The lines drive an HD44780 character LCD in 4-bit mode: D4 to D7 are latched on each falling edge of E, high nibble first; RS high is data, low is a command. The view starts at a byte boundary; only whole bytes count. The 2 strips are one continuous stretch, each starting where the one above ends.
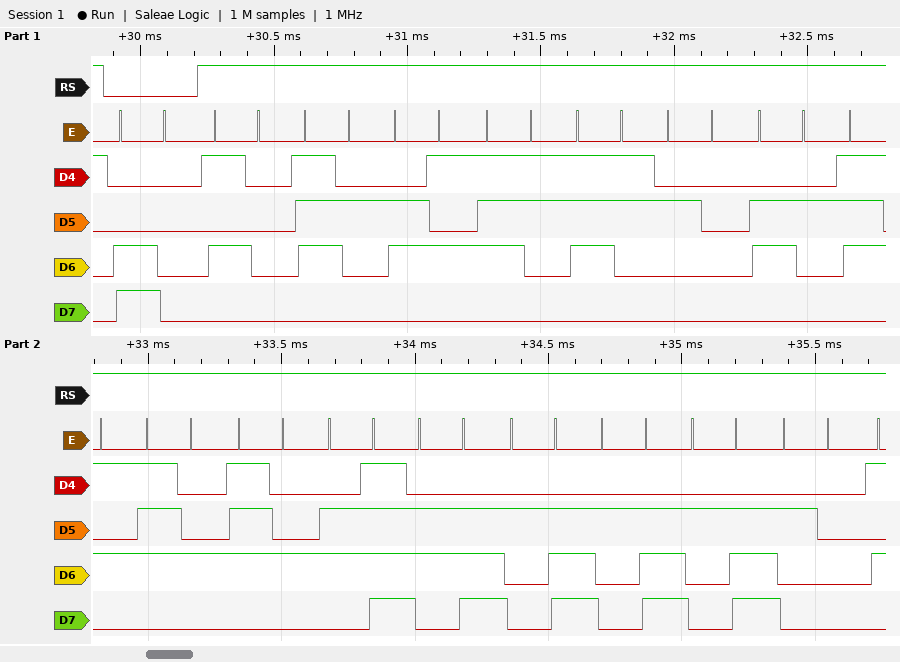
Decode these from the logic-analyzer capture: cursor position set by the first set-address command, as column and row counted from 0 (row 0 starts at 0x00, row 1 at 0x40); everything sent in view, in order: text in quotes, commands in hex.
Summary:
column 0, row 1
0xC0 "Press button... "
